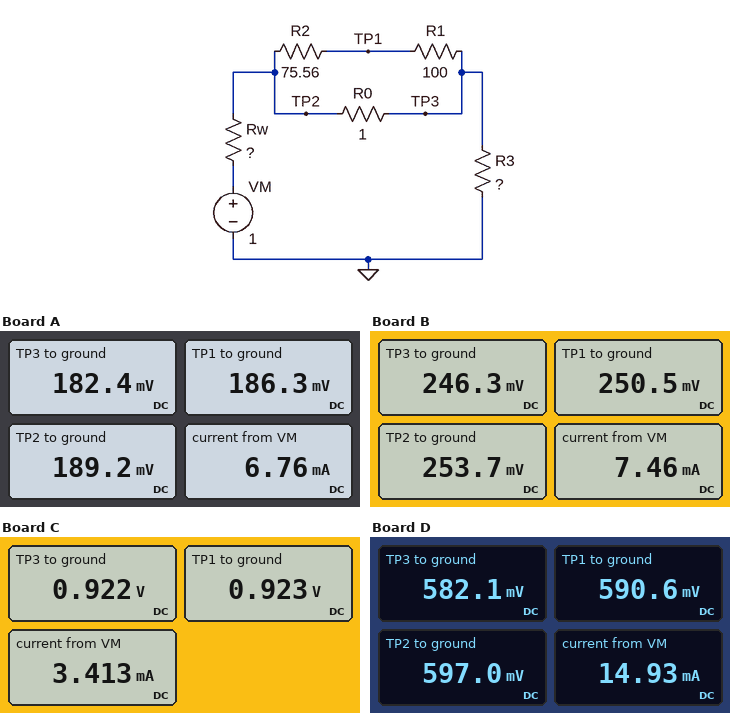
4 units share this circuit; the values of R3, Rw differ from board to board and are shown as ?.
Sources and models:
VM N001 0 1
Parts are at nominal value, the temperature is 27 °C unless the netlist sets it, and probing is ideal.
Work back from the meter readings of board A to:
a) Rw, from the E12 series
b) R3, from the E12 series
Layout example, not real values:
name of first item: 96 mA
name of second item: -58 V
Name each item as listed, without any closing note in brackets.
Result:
Rw, from the E12 series: 120 Ω
R3, from the E12 series: 27 Ω
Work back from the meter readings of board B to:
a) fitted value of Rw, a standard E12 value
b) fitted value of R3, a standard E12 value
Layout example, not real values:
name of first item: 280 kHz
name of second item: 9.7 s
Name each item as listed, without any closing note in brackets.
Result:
fitted value of Rw, a standard E12 value: 100 Ω
fitted value of R3, a standard E12 value: 33 Ω
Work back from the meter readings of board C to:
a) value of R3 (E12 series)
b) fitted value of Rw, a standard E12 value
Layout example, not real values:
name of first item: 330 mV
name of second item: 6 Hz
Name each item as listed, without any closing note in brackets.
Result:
value of R3: 270 Ω
fitted value of Rw, a standard E12 value: 22 Ω
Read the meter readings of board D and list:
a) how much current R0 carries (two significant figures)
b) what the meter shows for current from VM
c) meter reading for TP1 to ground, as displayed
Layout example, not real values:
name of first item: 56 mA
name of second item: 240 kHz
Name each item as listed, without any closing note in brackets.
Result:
how much current R0 carries: 15 mA
what the meter shows for current from VM: 14.93 mA
meter reading for TP1 to ground, as displayed: 590.6 mV
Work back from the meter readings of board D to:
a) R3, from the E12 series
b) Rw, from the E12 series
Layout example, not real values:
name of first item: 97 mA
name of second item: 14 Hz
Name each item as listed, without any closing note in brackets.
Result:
R3, from the E12 series: 39 Ω
Rw, from the E12 series: 27 Ω
